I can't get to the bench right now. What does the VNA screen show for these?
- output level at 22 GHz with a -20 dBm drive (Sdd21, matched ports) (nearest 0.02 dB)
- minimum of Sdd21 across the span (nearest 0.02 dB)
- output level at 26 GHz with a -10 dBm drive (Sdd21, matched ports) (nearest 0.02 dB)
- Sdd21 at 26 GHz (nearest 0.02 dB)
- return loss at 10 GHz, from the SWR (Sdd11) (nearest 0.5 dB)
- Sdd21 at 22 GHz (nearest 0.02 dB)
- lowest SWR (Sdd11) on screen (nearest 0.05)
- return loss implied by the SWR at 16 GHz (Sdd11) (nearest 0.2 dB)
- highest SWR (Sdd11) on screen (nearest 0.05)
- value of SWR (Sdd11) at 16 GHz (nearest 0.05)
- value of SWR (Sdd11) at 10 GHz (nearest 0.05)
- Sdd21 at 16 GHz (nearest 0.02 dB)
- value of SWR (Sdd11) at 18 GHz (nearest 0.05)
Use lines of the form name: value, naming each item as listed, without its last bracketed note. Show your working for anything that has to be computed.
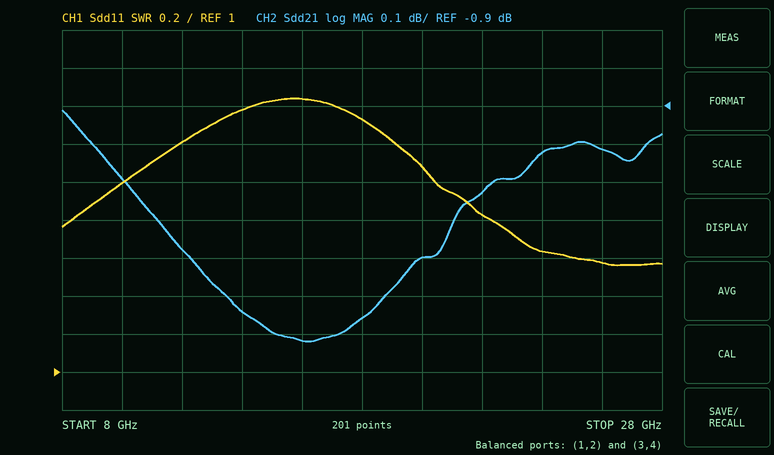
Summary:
output level at 22 GHz with a -20 dBm drive (Sdd21, matched ports): -20 dBm + (-1.12 dB) = -21.12 dBm
minimum of Sdd21 across the span: -1.52 dB
output level at 26 GHz with a -10 dBm drive (Sdd21, matched ports): -10 dBm + (-1.02 dB) = -11.02 dBm
Sdd21 at 26 GHz: -1.02 dB
return loss at 10 GHz, from the SWR (Sdd11): −20 log10((2 − 1)/(2 + 1)) ≈ 9.5 dB
Sdd21 at 22 GHz: -1.12 dB
lowest SWR (Sdd11) on screen: 1.55
return loss implied by the SWR at 16 GHz (Sdd11): −20 log10((2.45 − 1)/(2.45 + 1)) ≈ 7.53 dB, so 7.6 dB to the nearest 0.2 dB
highest SWR (Sdd11) on screen: 2.45
value of SWR (Sdd11) at 16 GHz: 2.45
value of SWR (Sdd11) at 10 GHz: 2.00
Sdd21 at 16 GHz: -1.52 dB
value of SWR (Sdd11) at 18 GHz: 2.35
